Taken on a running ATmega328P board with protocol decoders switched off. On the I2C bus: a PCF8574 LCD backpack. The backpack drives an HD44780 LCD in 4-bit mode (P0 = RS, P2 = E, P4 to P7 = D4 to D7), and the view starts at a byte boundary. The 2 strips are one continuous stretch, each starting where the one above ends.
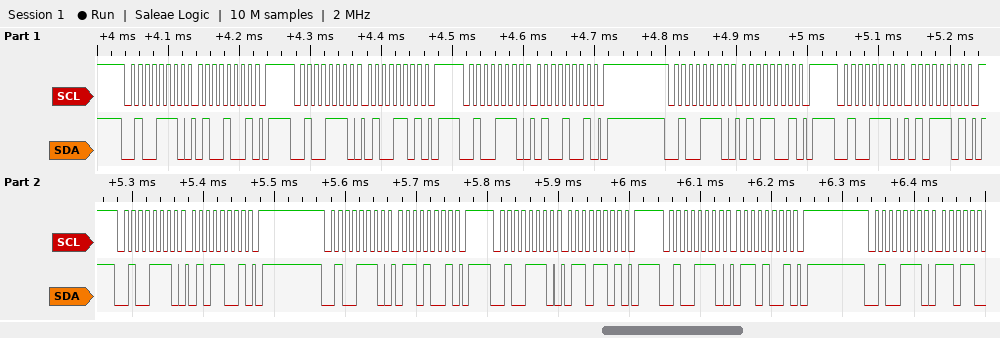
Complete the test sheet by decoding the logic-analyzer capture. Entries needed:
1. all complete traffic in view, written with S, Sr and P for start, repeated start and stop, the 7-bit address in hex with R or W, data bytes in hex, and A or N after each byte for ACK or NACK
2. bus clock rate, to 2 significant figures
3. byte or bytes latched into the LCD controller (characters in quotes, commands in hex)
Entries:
S 27W A 49 A P S 27W A 4D A P S 27W A 49 A P S 27W A 59 A P S 27W A 5D A P S 27W A 59 A P S 27W A 69 A P S 27W A 6D A P S 27W A 69 A P S 27W A
100 kHz
'E'
